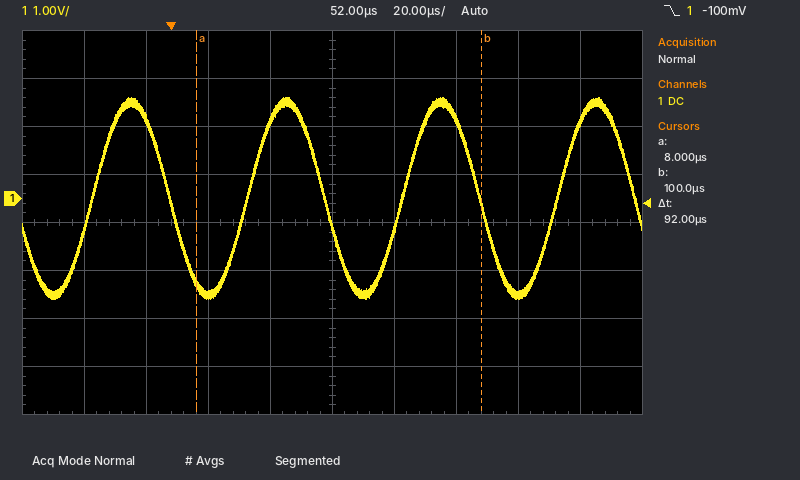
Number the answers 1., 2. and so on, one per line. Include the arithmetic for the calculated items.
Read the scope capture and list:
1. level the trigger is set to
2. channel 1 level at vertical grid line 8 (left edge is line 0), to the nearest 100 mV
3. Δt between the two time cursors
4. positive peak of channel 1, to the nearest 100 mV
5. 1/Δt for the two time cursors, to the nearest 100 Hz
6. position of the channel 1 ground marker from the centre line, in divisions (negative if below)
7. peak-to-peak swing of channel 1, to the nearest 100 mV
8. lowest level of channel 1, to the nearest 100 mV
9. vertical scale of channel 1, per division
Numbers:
1. -100 mV
2. -2.0 V
3. 92 µs
4. 2.1 V
5. 1 / 92 µs ≈ 10.9 kHz
6. +0.5 div
7. 2.1 V − (-2.1 V) = 4.2 V
8. -2.1 V
9. 1 V
